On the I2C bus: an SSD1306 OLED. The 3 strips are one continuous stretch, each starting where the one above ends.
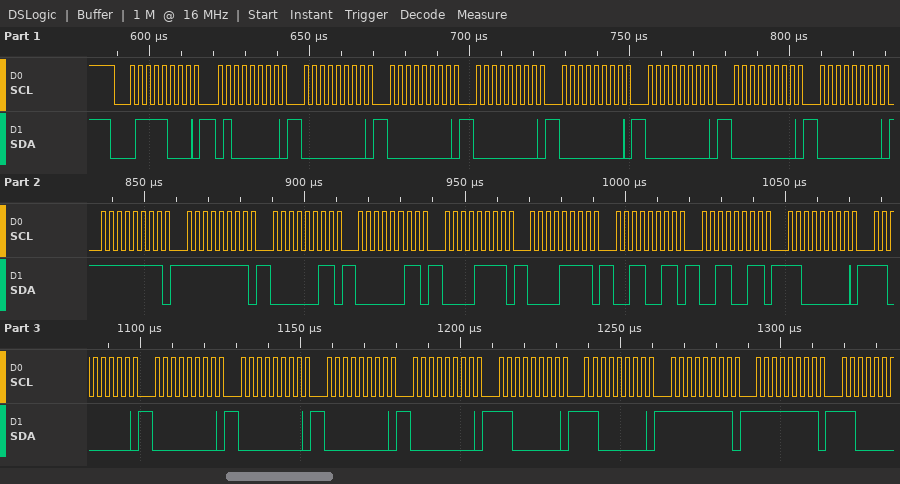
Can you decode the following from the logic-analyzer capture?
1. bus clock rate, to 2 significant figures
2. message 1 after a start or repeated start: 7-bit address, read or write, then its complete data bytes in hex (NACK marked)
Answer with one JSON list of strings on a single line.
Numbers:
["400 kHz", "0x3C write: 40 00 00 00 00 00 00 00 FF FF 03 03 0F 0F 33 33 C0 C0 00 00 00 00 C0 C0 FF FF"]
